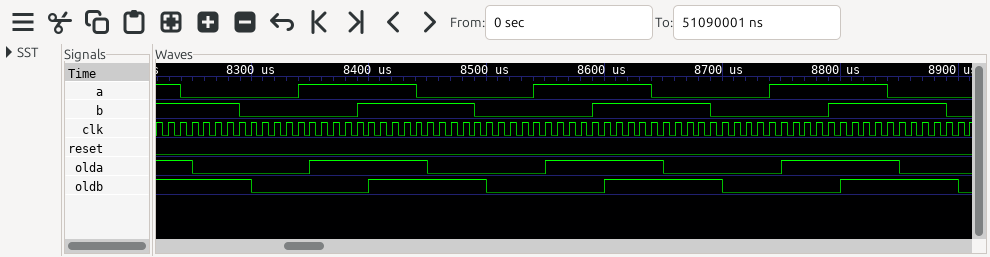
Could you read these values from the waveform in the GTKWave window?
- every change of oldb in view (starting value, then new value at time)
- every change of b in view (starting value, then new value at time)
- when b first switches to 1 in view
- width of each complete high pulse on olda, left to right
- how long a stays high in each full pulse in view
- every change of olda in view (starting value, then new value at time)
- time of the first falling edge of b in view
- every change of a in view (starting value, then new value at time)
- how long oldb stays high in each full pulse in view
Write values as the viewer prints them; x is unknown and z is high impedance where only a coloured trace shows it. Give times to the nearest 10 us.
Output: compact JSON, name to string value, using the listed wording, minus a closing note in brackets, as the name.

{"every change of oldb in view": "1, 0 at 8300 us, 1 at 8400 us, 0 at 8500 us, 1 at 8600 us, 0 at 8700 us, 1 at 8800 us, 0 at 8900 us", "every change of b in view": "1, 0 at 8290 us, 1 at 8390 us, 0 at 8490 us, 1 at 8590 us, 0 at 8690 us, 1 at 8790 us, 0 at 8890 us", "when b first switches to 1 in view": "8390 us", "width of each complete high pulse on olda, left to right": "100 us, 100 us, 100 us", "how long a stays high in each full pulse in view": "100 us, 100 us, 100 us", "every change of olda in view": "1, 0 at 8250 us, 1 at 8350 us, 0 at 8450 us, 1 at 8550 us, 0 at 8650 us, 1 at 8750 us, 0 at 8850 us", "time of the first falling edge of b in view": "8290 us", "every change of a in view": "1, 0 at 8240 us, 1 at 8340 us, 0 at 8440 us, 1 at 8540 us, 0 at 8640 us, 1 at 8740 us, 0 at 8840 us", "how long oldb stays high in each full pulse in view": "100 us, 100 us, 100 us"}
